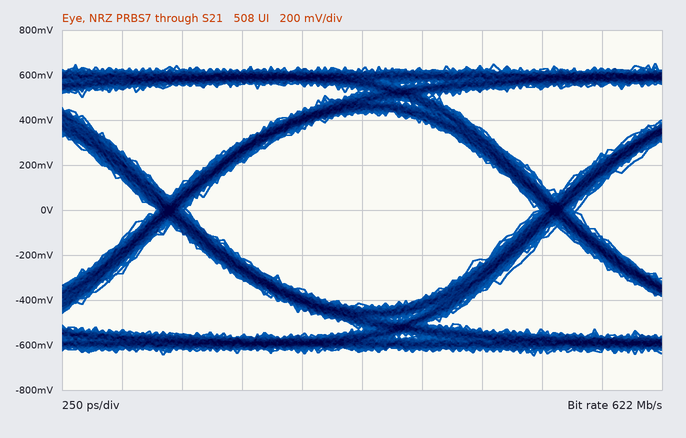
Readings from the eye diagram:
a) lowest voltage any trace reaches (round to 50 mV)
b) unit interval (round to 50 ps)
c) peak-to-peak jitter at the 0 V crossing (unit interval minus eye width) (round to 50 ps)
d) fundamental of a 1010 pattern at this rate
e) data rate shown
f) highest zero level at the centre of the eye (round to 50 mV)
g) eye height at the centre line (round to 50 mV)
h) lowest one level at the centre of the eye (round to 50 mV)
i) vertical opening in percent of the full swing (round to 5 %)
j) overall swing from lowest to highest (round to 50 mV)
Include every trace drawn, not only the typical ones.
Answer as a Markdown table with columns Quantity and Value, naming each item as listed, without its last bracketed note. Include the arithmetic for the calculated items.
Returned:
| Quantity | Value |
|---|---|
| lowest voltage any trace reaches | -650 mV |
| unit interval | 1.60 ns |
| peak-to-peak jitter at the 0 V crossing (unit interval minus eye width) | 150 ps |
| fundamental of a 1010 pattern at this rate | 311 MHz |
| data rate shown | 622 Mb/s |
| highest zero level at the centre of the eye | -400 mV |
| eye height at the centre line | 850 mV |
| lowest one level at the centre of the eye | 450 mV |
| vertical opening in percent of the full swing | 850 mV / 1.30 V ≈ 65 % |
| overall swing from lowest to highest | 1.30 V |
